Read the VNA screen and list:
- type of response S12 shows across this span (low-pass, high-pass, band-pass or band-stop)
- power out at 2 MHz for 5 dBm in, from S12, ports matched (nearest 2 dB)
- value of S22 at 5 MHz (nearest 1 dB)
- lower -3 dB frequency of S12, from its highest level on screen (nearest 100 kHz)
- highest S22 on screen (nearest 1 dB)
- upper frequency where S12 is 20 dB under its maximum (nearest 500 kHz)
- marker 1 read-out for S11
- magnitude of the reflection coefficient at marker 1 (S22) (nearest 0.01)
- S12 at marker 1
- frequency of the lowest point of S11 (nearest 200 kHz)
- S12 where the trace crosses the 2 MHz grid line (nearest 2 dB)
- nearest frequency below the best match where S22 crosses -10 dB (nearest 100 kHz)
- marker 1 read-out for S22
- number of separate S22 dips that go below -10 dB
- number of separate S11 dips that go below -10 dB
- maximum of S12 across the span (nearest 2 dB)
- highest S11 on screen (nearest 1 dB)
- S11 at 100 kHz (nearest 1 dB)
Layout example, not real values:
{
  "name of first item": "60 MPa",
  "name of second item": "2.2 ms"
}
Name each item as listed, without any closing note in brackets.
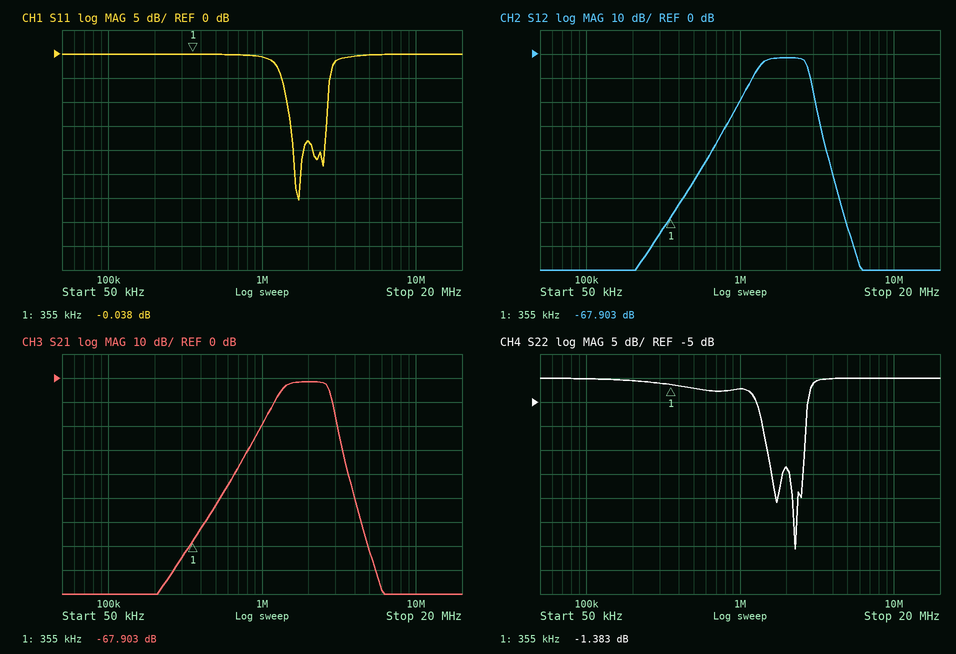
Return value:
{
  "type of response S12 shows across this span": "band-pass",
  "power out at 2 MHz for 5 dBm in, from S12, ports matched": "4 dBm",
  "value of S22 at 5 MHz": "0 dB",
  "lower -3 dB frequency of S12, from its highest level on screen": "1.4 MHz",
  "highest S22 on screen": "0 dB",
  "upper frequency where S12 is 20 dB under its maximum": "3.0 MHz",
  "marker 1 read-out for S11": "-0.038 dB",
  "magnitude of the reflection coefficient at marker 1 (S22)": "0.85",
  "S12 at marker 1": "-67.903 dB",
  "frequency of the lowest point of S11": "1.8 MHz",
  "S12 where the trace crosses the 2 MHz grid line": "-2 dB",
  "nearest frequency below the best match where S22 crosses -10 dB": "1.4 MHz",
  "marker 1 read-out for S22": "-1.383 dB",
  "number of separate S22 dips that go below -10 dB": "2",
  "number of separate S11 dips that go below -10 dB": "2",
  "maximum of S12 across the span": "-2 dB",
  "highest S11 on screen": "0 dB",
  "S11 at 100 kHz": "0 dB"
}
